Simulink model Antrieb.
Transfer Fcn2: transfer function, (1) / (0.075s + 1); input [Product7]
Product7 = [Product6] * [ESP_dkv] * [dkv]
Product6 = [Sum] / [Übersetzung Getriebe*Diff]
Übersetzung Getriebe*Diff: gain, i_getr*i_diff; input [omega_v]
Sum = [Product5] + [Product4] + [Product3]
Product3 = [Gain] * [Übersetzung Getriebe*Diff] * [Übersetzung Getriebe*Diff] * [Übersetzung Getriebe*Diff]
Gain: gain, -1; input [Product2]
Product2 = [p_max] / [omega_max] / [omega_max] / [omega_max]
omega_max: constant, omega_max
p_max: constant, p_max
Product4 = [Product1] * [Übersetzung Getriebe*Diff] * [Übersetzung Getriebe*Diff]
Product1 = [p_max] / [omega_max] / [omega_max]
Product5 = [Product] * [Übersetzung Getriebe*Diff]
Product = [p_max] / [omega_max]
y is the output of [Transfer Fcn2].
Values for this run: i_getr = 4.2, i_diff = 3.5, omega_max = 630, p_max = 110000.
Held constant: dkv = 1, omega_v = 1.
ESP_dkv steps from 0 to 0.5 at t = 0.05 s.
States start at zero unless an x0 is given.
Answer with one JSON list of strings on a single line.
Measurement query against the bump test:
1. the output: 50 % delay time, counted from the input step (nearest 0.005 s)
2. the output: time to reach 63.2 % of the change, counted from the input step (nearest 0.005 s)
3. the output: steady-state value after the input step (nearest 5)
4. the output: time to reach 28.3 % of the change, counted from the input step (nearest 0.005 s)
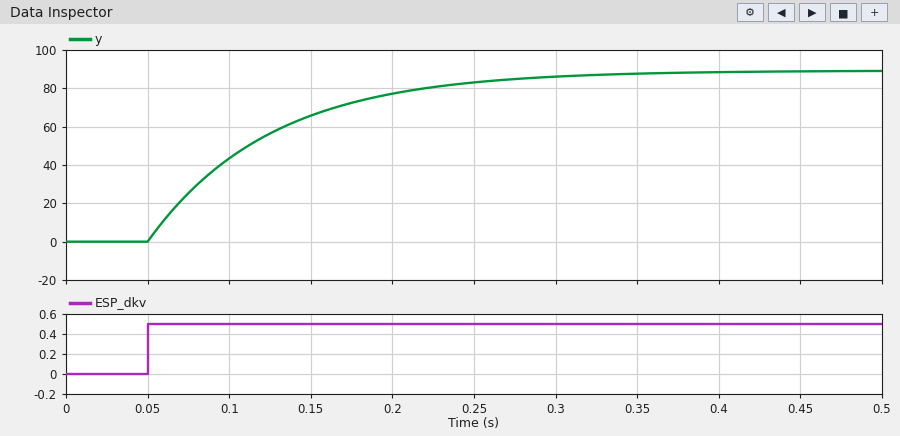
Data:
["0.050 s", "0.075 s", "90", "0.025 s"]
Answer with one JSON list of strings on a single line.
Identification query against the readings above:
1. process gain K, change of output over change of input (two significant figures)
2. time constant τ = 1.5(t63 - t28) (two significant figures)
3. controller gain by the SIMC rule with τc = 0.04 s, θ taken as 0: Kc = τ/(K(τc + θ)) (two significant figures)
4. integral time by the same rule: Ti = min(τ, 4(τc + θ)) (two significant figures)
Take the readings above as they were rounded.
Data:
["180", "0.075 s", "0.010", "0.075 s"]
